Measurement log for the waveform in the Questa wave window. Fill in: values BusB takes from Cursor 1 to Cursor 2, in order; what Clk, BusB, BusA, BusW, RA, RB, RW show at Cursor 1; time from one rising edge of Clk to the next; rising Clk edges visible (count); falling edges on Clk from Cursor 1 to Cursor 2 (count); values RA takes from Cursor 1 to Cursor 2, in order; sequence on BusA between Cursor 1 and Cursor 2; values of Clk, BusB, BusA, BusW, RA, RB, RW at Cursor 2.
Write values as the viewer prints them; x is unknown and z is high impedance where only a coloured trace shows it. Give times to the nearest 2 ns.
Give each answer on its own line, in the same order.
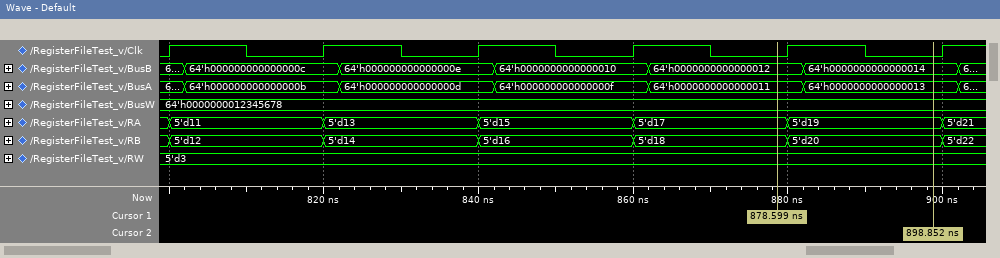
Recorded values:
64'h0000000000000012, 64'h0000000000000014
Clk=0, BusB=64'h0000000000000012, BusA=64'h0000000000000011, BusW=64'h0000000012345678, RA=5'd17, RB=5'd18, RW=5'd3
20 ns
6
1
5'd17, 5'd19
64'h0000000000000011, 64'h0000000000000013
Clk=0, BusB=64'h0000000000000014, BusA=64'h0000000000000013, BusW=64'h0000000012345678, RA=5'd19, RB=5'd20, RW=5'd3
